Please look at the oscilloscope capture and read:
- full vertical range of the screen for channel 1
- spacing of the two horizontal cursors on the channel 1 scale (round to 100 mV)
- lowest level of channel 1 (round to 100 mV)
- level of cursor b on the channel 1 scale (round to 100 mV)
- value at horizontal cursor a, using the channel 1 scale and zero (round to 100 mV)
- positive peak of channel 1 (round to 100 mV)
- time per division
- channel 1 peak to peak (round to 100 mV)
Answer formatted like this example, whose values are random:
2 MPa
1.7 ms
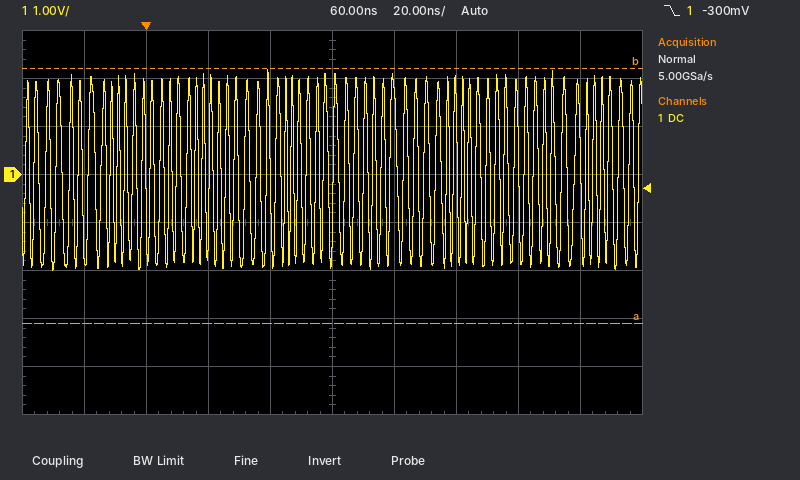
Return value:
8 V
5.3 V
-2.0 V
2.2 V
-3.1 V
2.2 V
20 ns
4.2 V
